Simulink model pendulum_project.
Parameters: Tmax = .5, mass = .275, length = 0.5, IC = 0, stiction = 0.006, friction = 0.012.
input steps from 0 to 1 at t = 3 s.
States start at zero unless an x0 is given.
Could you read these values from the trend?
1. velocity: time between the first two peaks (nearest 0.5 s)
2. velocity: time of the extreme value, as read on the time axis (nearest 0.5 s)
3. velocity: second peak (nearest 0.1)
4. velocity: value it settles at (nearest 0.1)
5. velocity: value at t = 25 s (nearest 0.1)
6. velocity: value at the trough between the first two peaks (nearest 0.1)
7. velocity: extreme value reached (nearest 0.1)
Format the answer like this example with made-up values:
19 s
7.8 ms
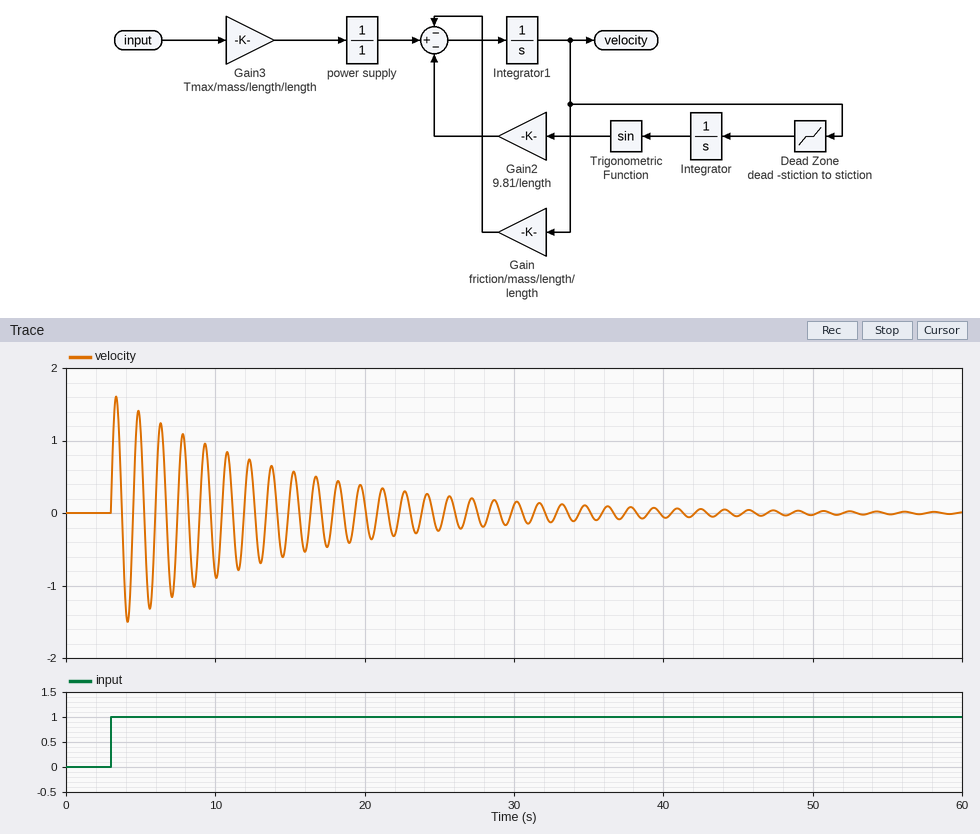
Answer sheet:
1.5 s
3.5 s
1.4
0.0
-0.2
-1.5
1.6
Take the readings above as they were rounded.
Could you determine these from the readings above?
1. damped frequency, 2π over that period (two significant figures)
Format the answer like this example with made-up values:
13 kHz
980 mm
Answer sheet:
4.2 rad/s
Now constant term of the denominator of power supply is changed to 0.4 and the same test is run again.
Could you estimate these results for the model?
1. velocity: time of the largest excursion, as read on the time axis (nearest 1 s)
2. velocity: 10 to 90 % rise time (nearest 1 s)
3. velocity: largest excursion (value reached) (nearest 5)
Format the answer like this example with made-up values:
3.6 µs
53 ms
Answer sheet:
60 s
10 s
105
